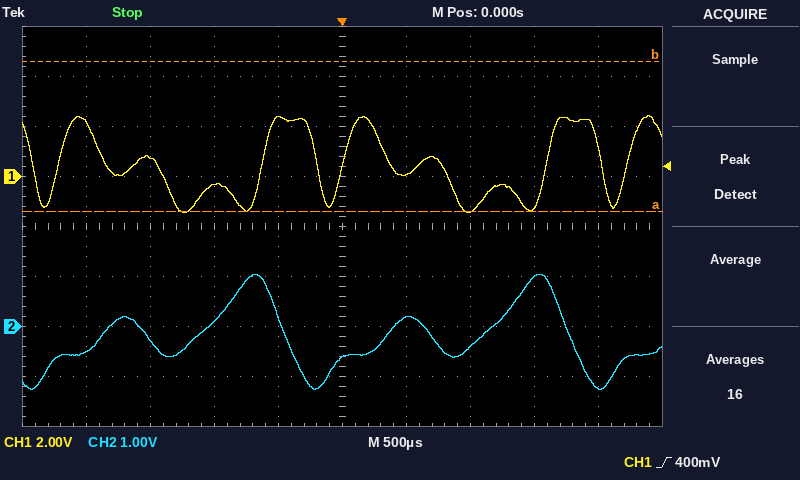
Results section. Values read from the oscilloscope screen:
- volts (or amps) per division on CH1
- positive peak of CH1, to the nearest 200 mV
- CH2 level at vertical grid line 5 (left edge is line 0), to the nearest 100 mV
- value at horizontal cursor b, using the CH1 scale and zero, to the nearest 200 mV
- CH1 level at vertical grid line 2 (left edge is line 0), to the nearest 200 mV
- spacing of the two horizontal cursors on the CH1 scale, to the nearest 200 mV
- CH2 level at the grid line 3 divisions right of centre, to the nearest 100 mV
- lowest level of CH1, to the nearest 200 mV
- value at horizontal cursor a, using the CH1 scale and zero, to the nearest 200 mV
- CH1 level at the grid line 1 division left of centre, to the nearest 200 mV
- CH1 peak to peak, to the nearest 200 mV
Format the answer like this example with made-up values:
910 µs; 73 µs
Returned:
2 V; 2.4 V; -600 mV; 4.6 V; 800 mV; 6.0 V; 1.0 V; -1.4 V; -1.4 V; 2.4 V; 3.8 V
